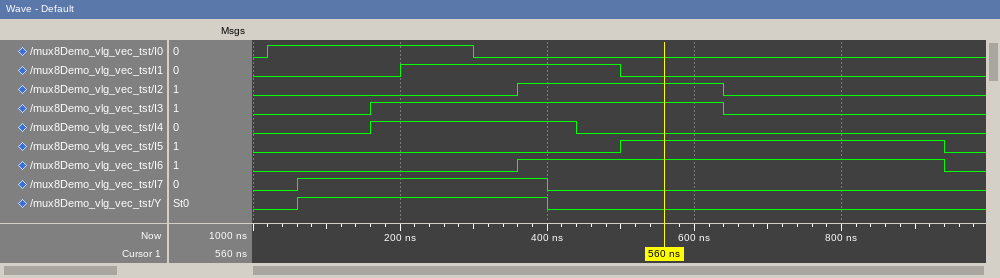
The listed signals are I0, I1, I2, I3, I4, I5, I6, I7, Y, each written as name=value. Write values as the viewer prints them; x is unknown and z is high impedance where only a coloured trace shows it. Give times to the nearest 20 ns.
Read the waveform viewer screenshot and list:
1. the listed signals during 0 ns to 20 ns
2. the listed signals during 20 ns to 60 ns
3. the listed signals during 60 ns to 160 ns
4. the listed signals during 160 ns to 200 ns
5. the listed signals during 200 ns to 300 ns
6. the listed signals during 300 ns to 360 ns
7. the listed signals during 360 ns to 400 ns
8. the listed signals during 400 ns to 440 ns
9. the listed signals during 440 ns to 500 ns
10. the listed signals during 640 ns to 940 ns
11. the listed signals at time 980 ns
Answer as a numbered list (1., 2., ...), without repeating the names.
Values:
1. I0=0, I1=0, I2=0, I3=0, I4=0, I5=0, I6=0, I7=0, Y=0
2. I0=1, I1=0, I2=0, I3=0, I4=0, I5=0, I6=0, I7=0, Y=0
3. I0=1, I1=0, I2=0, I3=0, I4=0, I5=0, I6=0, I7=1, Y=1
4. I0=1, I1=0, I2=0, I3=1, I4=1, I5=0, I6=0, I7=1, Y=1
5. I0=1, I1=1, I2=0, I3=1, I4=1, I5=0, I6=0, I7=1, Y=1
6. I0=0, I1=1, I2=0, I3=1, I4=1, I5=0, I6=0, I7=1, Y=1
7. I0=0, I1=1, I2=1, I3=1, I4=1, I5=0, I6=1, I7=1, Y=1
8. I0=0, I1=1, I2=1, I3=1, I4=1, I5=0, I6=1, I7=0, Y=0
9. I0=0, I1=1, I2=1, I3=1, I4=0, I5=0, I6=1, I7=0, Y=0
10. I0=0, I1=0, I2=0, I3=0, I4=0, I5=1, I6=1, I7=0, Y=0
11. I0=0, I1=0, I2=0, I3=0, I4=0, I5=0, I6=0, I7=0, Y=0
